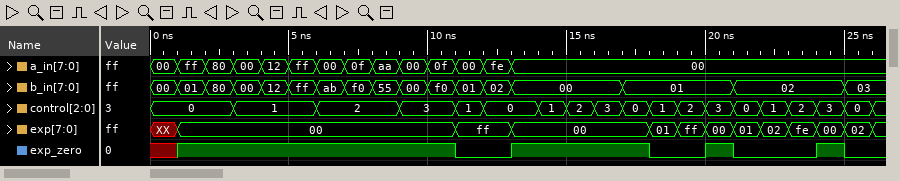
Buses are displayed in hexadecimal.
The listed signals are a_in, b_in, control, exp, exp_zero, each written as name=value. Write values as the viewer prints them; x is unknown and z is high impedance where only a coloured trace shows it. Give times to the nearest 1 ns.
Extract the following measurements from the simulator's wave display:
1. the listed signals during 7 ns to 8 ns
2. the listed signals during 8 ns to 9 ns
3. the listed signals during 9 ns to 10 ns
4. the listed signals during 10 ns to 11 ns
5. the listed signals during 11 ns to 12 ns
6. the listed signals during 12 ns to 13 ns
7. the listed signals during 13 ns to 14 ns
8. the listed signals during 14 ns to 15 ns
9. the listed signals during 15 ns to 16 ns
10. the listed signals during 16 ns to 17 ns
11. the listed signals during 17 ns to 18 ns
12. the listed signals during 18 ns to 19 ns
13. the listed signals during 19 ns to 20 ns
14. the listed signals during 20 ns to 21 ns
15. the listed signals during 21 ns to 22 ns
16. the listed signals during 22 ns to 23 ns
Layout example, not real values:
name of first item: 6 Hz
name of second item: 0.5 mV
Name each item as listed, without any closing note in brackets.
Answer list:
the listed signals during 7 ns to 8 ns: a_in=0f, b_in=f0, control=2, exp=00, exp_zero=1
the listed signals during 8 ns to 9 ns: a_in=aa, b_in=55, control=2, exp=00, exp_zero=1
the listed signals during 9 ns to 10 ns: a_in=00, b_in=00, control=3, exp=00, exp_zero=1
the listed signals during 10 ns to 11 ns: a_in=0f, b_in=f0, control=3, exp=00, exp_zero=1
the listed signals during 11 ns to 12 ns: a_in=00, b_in=01, control=1, exp=ff, exp_zero=0
the listed signals during 12 ns to 13 ns: a_in=fe, b_in=02, control=0, exp=ff, exp_zero=0
the listed signals during 13 ns to 14 ns: a_in=00, b_in=00, control=0, exp=00, exp_zero=1
the listed signals during 14 ns to 15 ns: a_in=00, b_in=00, control=1, exp=00, exp_zero=1
the listed signals during 15 ns to 16 ns: a_in=00, b_in=00, control=2, exp=00, exp_zero=1
the listed signals during 16 ns to 17 ns: a_in=00, b_in=00, control=3, exp=00, exp_zero=1
the listed signals during 17 ns to 18 ns: a_in=00, b_in=01, control=0, exp=00, exp_zero=1
the listed signals during 18 ns to 19 ns: a_in=00, b_in=01, control=1, exp=01, exp_zero=0
the listed signals during 19 ns to 20 ns: a_in=00, b_in=01, control=2, exp=ff, exp_zero=0
the listed signals during 20 ns to 21 ns: a_in=00, b_in=01, control=3, exp=00, exp_zero=1
the listed signals during 21 ns to 22 ns: a_in=00, b_in=02, control=0, exp=01, exp_zero=0
the listed signals during 22 ns to 23 ns: a_in=00, b_in=02, control=1, exp=02, exp_zero=0
